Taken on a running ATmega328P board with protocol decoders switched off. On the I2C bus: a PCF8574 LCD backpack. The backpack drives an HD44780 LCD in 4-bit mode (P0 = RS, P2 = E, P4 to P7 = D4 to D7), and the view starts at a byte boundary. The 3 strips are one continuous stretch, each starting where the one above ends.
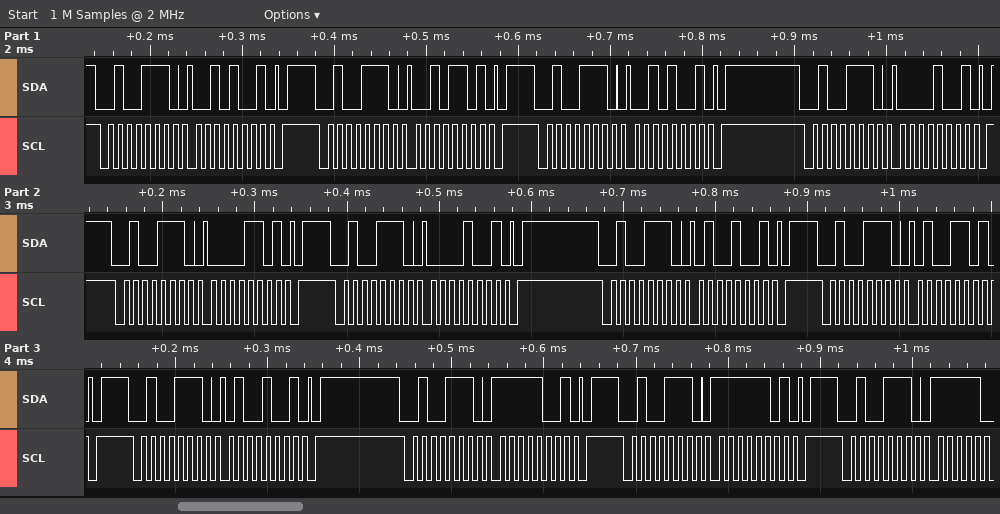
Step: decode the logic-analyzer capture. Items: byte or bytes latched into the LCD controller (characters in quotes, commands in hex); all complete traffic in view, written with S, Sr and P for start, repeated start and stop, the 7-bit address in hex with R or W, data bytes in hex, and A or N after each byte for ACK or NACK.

' '
S 27W A 29 A P S 27W A 2D A P S 27W A 29 A P S 27W A 09 A P S 27W A 0D A P S 27W A 09 A P S 27W A 49 A P S 27W A 4D A P S 27W A 49 A P S 27W A F9 A P S 27W A FD A P S 27W A
